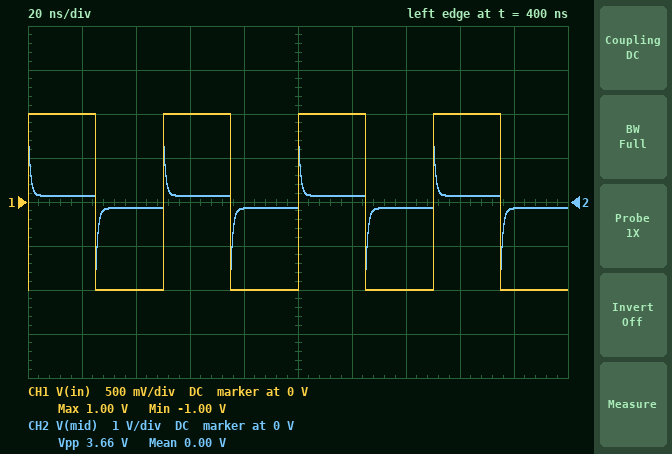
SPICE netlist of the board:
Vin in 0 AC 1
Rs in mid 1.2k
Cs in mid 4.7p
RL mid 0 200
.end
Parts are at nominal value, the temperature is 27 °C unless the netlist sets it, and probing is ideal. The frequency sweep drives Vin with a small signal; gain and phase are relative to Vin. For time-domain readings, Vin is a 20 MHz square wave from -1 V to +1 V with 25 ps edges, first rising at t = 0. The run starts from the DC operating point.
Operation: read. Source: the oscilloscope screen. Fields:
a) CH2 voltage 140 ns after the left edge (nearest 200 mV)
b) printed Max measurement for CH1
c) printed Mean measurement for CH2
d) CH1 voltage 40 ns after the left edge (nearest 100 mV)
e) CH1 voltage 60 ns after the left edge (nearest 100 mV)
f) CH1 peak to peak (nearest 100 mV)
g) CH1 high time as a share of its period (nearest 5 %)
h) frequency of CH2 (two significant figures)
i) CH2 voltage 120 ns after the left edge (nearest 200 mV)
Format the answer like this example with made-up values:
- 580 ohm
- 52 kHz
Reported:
- -200 mV
- 1.00 V
- 0.00 V
- -1.0 V
- 1.0 V
- 2.0 V
- 50 %
- 20 MHz
- 200 mV
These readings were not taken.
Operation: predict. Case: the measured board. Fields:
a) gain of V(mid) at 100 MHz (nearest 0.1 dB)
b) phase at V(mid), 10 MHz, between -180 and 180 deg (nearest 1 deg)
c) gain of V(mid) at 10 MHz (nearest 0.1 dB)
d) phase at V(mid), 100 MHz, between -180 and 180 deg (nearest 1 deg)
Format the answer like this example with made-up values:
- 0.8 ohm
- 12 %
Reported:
- -6.6 dB
- 17 deg
- -16.4 dB
- 47 deg
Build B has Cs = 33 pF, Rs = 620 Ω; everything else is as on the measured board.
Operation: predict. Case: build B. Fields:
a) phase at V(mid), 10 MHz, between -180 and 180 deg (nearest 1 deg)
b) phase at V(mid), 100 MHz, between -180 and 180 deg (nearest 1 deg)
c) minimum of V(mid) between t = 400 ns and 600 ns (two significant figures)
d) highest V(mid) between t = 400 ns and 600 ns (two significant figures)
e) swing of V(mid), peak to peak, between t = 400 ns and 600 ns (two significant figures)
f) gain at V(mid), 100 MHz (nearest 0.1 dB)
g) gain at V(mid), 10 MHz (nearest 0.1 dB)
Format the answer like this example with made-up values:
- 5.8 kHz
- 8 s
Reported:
- 35 deg
- 13 deg
- -1.7 V
- 1.7 V
- 3.5 V
- -0.4 dB
- -8.4 dB
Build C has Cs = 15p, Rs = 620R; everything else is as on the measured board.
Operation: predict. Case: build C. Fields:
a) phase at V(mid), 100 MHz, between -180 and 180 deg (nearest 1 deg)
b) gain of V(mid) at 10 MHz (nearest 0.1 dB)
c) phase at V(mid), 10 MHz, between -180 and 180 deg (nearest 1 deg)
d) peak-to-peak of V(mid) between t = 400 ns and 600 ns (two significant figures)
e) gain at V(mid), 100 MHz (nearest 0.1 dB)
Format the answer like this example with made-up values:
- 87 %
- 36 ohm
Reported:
- 25 deg
- -11.1 dB
- 22 deg
- 3.5 V
- -1.6 dB
